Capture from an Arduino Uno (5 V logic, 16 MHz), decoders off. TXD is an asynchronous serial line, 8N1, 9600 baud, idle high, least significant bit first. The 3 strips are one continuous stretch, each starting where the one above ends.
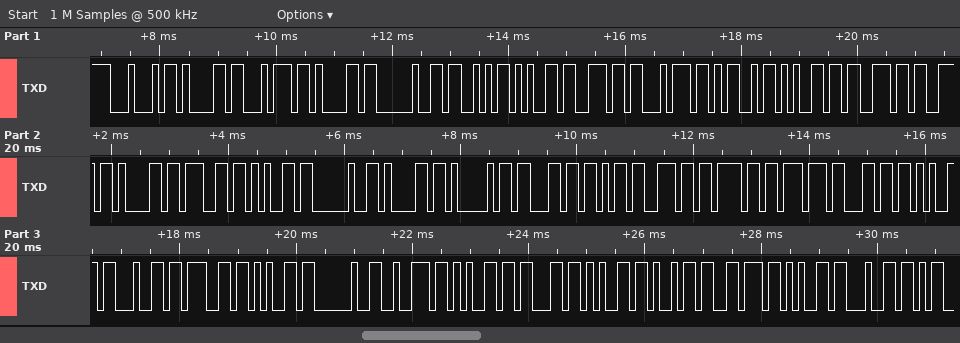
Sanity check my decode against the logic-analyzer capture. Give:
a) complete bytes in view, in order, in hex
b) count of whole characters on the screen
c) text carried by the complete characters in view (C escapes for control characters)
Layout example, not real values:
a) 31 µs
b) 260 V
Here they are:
a) 44 61 74 61 20 53 65 6E 74 4D 65 73 73 61 67 65 20 61 41 63 6B 6E 6F 77 6C 65 64 67 65 20 72 65 63 65 69 76 65 64
b) 38
c) "Data SentMessage aAcknowledge received"
